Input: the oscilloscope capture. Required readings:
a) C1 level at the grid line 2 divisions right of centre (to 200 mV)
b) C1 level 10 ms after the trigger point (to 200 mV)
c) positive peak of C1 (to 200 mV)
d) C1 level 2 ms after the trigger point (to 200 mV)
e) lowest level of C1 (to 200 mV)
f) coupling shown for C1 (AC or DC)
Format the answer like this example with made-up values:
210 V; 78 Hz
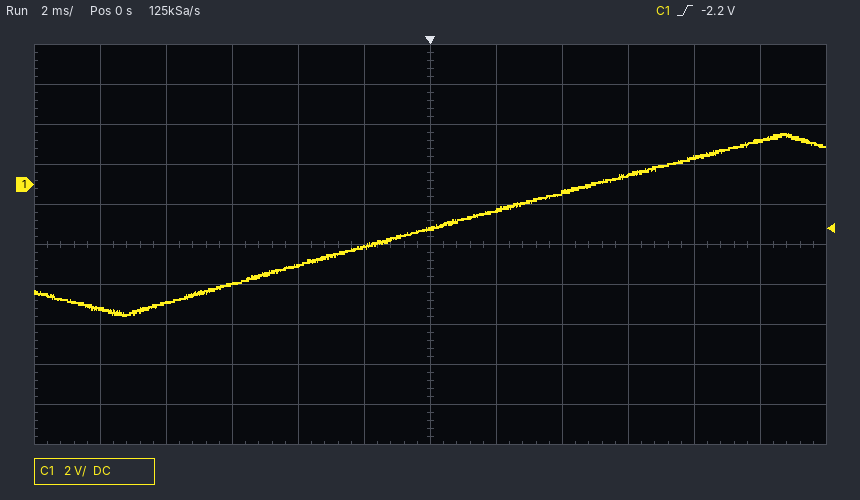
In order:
-400 mV; 2.2 V; 2.6 V; -1.2 V; -6.6 V; DC
